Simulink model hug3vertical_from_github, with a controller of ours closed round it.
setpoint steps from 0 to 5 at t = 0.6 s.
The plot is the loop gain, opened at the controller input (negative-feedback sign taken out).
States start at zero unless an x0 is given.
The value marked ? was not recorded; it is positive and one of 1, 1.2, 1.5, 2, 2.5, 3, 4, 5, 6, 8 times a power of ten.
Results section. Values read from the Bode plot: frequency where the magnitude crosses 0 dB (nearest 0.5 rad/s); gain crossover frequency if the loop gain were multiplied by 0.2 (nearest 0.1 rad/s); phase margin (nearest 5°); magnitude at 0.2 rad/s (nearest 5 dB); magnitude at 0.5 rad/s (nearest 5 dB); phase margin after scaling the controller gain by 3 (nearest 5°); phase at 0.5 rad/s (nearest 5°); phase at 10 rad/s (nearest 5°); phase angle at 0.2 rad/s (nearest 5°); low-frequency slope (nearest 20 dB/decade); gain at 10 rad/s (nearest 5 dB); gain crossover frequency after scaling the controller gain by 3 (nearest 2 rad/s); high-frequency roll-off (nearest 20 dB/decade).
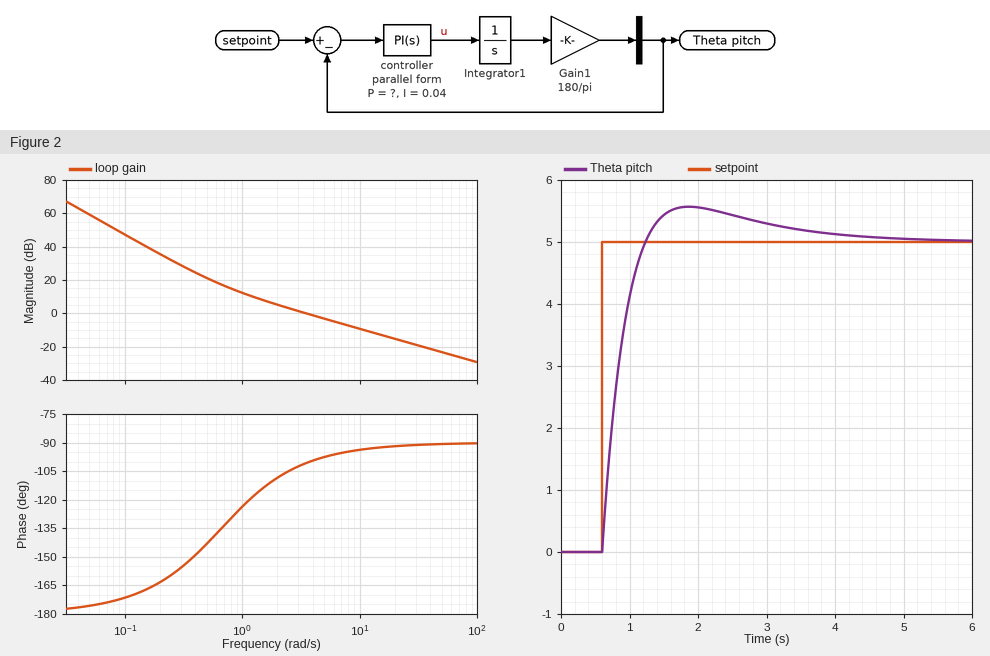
3.5 rad/s
0.9 rad/s
80°
35 dB
20 dB
85°
-145°
-95°
-165°
-40 dB/decade
-10 dB
10 rad/s
-20 dB/decade
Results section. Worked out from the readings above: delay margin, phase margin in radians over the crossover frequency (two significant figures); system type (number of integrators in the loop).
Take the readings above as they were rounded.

0.40 s
2
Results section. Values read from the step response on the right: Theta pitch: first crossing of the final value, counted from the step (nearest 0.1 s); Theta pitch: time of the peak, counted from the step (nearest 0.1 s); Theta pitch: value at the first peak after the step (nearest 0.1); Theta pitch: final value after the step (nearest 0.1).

0.6 s
1.3 s
5.6
5.0
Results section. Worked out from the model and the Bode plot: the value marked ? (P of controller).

0.06
